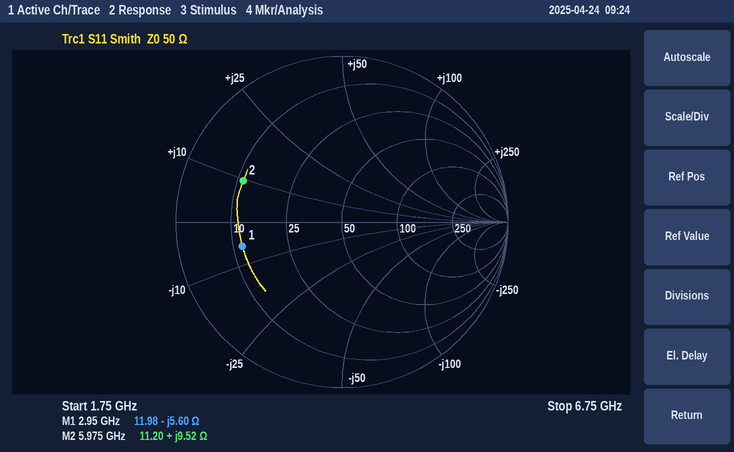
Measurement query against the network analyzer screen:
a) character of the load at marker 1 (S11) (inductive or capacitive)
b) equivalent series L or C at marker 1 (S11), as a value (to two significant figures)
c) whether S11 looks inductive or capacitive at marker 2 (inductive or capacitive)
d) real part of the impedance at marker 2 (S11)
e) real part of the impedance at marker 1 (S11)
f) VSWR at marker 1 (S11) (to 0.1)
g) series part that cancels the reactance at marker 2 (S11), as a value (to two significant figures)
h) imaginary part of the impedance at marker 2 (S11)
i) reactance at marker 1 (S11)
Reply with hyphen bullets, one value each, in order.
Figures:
- capacitive
- 9.6 pF
- inductive
- 11.20 Ω
- 11.98 Ω
- 4.2
- 2.8 pF
- +9.52 Ω
- -5.60 Ω
